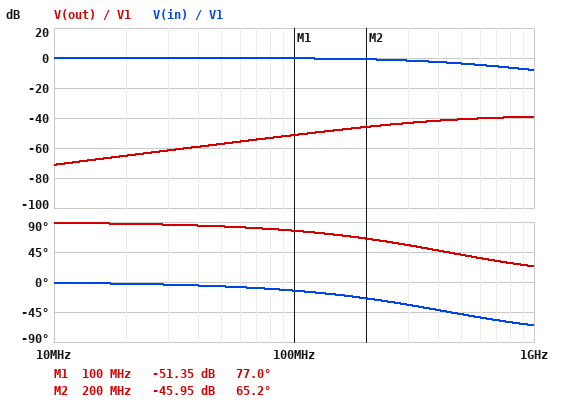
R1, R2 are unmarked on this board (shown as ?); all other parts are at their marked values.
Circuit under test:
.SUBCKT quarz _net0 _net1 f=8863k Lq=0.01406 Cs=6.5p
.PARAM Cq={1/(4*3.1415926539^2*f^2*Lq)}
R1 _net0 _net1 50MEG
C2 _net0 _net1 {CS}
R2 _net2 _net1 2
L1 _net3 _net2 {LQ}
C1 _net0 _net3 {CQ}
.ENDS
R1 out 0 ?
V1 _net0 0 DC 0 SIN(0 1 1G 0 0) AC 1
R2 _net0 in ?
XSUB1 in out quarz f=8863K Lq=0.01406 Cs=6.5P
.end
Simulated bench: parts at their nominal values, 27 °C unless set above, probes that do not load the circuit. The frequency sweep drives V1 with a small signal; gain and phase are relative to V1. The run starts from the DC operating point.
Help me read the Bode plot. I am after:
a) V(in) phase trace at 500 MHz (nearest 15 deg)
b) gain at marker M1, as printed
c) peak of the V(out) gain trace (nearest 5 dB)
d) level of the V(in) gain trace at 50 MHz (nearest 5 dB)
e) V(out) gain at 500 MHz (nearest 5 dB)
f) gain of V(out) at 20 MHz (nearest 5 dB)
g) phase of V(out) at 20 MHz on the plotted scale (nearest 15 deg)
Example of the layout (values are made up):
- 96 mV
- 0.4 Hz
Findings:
- -45 deg
- -51.35 dB
- -40 dB
- 0 dB
- -40 dB
- -65 dB
- 90 deg
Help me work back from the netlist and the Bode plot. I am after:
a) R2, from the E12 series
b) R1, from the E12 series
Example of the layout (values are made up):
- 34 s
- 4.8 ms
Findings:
- 56 Ω
- 0.68 Ω
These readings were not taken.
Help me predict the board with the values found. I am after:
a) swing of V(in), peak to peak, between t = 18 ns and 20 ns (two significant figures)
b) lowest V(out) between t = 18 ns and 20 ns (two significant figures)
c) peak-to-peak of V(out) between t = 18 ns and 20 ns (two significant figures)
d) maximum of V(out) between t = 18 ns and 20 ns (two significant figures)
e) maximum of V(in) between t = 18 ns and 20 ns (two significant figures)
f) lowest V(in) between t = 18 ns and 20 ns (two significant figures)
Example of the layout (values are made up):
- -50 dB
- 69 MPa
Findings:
- 790 mV
- -11 mV
- 22 mV
- 11 mV
- 400 mV
- -400 mV
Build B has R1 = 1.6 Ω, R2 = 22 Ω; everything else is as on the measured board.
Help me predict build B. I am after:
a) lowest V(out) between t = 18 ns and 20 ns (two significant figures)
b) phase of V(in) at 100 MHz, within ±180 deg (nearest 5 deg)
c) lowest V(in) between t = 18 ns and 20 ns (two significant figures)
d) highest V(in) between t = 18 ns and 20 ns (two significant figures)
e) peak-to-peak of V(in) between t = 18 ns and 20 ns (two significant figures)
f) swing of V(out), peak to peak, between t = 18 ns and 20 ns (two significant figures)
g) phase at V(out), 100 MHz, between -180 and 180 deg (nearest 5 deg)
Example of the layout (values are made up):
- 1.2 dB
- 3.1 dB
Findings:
- -47 mV
- -5 deg
- -720 mV
- 720 mV
- 1.4 V
- 94 mV
- 85 deg
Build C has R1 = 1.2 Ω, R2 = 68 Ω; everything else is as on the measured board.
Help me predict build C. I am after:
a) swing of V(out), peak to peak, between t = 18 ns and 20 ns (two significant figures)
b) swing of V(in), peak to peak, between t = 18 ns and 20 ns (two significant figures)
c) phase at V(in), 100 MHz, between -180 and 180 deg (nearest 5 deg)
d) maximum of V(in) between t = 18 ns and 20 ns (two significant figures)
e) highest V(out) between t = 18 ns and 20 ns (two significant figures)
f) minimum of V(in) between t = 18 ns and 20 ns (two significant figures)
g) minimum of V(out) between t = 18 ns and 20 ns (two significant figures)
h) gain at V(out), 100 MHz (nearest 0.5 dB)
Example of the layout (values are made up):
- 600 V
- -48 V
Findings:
- 33 mV
- 670 mV
- -15 deg
- 330 mV
- 16 mV
- -330 mV
- -16 mV
- -46.5 dB
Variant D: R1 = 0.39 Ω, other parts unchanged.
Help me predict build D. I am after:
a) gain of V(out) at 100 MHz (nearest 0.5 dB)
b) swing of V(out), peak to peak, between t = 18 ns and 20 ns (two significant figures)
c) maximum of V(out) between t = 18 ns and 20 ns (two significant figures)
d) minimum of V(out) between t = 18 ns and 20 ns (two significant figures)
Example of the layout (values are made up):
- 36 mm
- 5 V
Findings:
- -56.0 dB
- 13 mV
- 6.3 mV
- -6.3 mV
